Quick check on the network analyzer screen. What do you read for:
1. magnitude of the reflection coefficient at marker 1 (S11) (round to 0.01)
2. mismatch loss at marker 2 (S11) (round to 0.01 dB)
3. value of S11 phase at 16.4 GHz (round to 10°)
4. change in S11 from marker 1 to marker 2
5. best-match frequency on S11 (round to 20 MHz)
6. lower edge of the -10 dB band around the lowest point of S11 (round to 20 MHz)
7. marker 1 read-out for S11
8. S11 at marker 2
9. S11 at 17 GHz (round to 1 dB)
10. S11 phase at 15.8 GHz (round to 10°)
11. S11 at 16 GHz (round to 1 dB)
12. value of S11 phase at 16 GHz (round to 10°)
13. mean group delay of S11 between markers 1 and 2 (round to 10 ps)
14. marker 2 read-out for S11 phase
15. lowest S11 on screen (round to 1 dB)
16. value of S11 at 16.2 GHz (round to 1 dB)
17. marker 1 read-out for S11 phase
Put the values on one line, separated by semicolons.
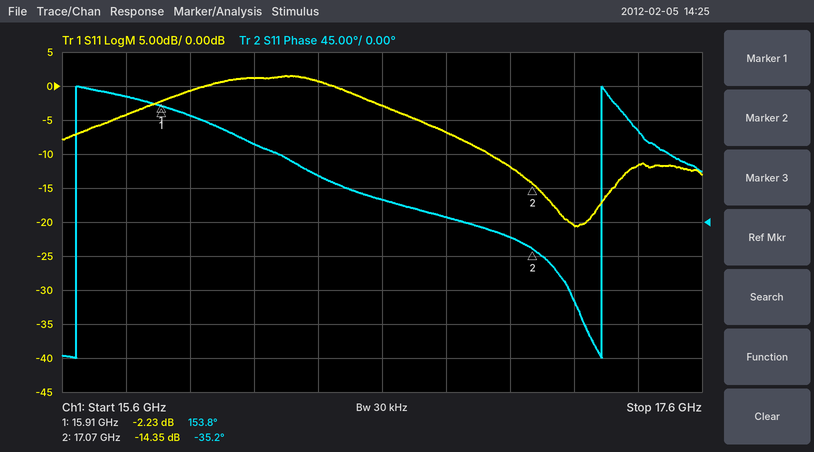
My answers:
0.77; 0.16 dB; 60°; -12.12 dB; 17.20 GHz; 16.94 GHz; -2.23 dB; -14.35 dB; -12 dB; 170°; -1 dB; 140°; 450 ps; -35.2°; -21 dB; 1 dB; 153.8°
